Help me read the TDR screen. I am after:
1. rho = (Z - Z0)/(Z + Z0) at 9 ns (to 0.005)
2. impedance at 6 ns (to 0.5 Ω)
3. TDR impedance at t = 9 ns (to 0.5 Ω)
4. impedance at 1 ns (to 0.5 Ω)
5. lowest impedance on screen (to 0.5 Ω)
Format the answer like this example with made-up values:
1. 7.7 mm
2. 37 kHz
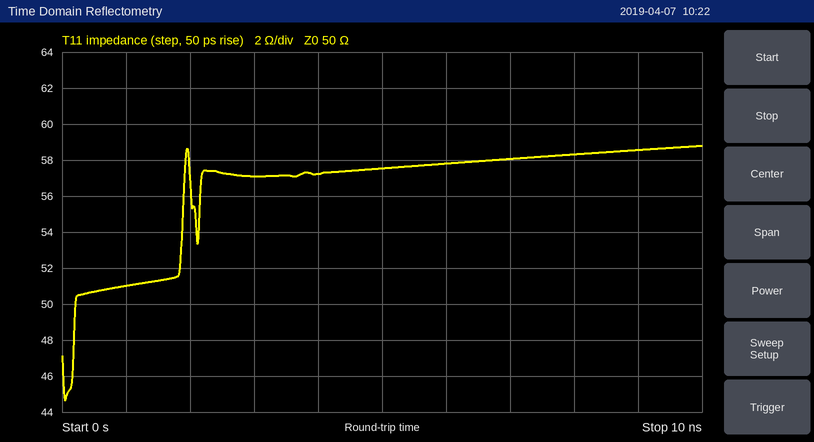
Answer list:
1. +0.080
2. 58.0 Ω
3. 58.5 Ω
4. 51.0 Ω
5. 44.5 Ω
